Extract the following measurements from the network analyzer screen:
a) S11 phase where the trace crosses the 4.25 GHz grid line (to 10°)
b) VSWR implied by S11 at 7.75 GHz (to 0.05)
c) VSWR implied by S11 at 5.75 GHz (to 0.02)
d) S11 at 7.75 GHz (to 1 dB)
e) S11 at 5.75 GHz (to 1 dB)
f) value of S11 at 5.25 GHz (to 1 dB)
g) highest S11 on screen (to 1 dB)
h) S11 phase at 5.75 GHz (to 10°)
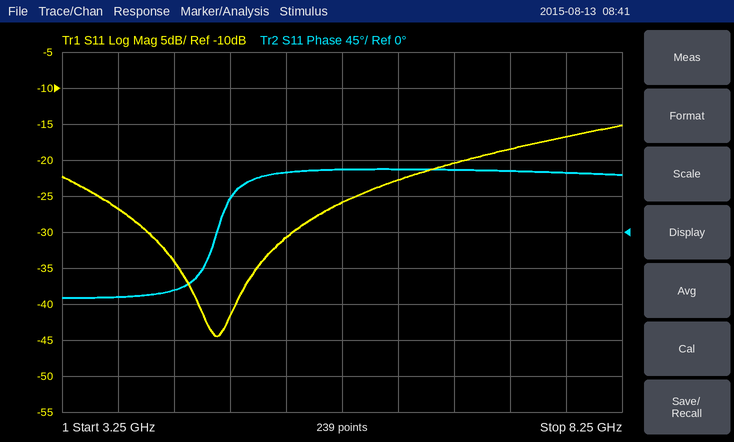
-70°
1.35
1.10
-17 dB
-26 dB
-31 dB
-15 dB
80°
